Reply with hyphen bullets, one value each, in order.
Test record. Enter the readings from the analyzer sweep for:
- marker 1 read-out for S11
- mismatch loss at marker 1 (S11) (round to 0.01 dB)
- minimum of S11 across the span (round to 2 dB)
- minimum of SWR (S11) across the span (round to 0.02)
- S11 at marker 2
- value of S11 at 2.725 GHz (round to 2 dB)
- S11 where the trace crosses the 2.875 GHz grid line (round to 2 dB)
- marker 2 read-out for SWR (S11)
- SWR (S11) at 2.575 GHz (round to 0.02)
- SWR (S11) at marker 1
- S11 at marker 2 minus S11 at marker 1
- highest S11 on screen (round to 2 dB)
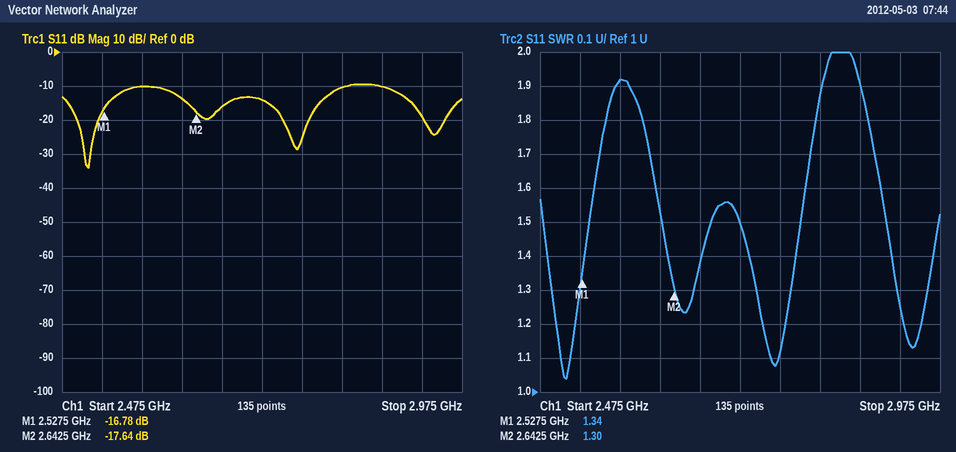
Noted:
- -16.78 dB
- 0.09 dB
- -34 dB
- 1.04
- -17.64 dB
- -14 dB
- -10 dB
- 1.30
- 1.92
- 1.34
- -0.86 dB
- -10 dB
